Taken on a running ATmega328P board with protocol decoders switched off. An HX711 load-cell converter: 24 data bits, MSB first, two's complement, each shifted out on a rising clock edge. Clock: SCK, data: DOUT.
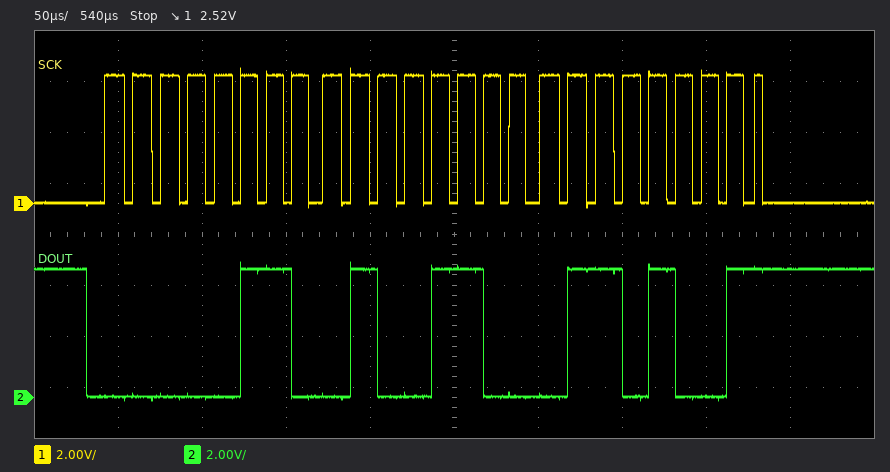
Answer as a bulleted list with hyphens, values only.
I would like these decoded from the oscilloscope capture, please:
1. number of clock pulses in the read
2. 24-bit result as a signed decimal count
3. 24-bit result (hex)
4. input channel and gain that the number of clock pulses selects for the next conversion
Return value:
- 25
- 412777
- 0x064C69
- channel A, gain 128
